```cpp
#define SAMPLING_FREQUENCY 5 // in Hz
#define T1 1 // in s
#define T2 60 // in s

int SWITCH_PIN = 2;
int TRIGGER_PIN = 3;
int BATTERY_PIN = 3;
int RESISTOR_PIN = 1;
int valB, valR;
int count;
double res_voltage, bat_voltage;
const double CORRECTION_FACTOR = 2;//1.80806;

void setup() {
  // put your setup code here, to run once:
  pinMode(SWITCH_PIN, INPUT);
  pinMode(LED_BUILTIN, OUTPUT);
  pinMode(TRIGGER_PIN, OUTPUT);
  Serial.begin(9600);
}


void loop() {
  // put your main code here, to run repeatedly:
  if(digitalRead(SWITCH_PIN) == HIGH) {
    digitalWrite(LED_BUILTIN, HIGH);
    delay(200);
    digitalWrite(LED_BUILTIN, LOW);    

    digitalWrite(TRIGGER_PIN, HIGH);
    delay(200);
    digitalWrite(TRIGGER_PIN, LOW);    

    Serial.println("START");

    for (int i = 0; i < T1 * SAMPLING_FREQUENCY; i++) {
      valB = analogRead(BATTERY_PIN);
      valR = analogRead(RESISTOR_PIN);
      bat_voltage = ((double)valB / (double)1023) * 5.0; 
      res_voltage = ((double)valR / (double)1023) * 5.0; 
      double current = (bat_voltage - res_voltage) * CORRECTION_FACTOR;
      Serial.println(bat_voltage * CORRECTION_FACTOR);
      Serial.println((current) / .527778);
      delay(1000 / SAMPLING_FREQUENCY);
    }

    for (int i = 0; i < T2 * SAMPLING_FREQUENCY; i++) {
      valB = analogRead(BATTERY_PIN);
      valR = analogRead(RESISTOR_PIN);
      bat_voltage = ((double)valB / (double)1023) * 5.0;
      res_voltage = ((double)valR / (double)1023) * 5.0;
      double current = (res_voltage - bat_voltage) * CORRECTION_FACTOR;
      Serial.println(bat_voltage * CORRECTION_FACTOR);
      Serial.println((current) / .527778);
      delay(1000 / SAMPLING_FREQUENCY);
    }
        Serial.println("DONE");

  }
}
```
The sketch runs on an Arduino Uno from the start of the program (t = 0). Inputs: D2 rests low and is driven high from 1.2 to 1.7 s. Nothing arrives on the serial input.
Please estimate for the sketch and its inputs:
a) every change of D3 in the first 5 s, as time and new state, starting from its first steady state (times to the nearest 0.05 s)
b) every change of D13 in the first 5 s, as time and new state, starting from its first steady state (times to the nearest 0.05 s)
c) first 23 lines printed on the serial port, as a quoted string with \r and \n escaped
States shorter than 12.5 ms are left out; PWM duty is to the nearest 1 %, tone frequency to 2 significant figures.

0 s low; 1.4 s high; 1.6 s low
0 s low; 1.2 s high; 1.4 s low
"START\r\n0.00\r\n0.00\r\n0.00\r\n0.00\r\n0.00\r\n0.00\r\n0.00\r\n0.00\r\n0.00\r\n0.00\r\n0.00\r\n0.00\r\n0.00\r\n0.00\r\n0.00\r\n0.00\r\n0.00\r\n0.00\r\n0.00\r\n0.00\r\n0.00\r\n0.00\r\n"
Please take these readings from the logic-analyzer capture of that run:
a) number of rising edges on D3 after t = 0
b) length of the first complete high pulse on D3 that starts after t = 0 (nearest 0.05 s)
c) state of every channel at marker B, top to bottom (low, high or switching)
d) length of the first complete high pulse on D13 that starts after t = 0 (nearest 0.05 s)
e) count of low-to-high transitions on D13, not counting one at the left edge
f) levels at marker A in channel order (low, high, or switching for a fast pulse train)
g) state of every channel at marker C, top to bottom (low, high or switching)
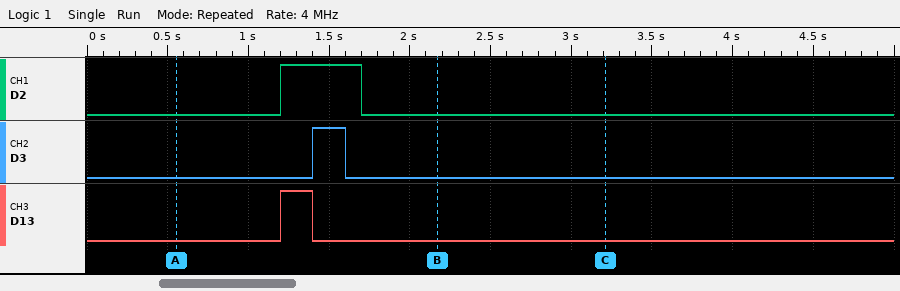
1
0.20 s
D2 low, D3 low, D13 low
0.20 s
1
D2 low, D3 low, D13 low
D2 low, D3 low, D13 low
